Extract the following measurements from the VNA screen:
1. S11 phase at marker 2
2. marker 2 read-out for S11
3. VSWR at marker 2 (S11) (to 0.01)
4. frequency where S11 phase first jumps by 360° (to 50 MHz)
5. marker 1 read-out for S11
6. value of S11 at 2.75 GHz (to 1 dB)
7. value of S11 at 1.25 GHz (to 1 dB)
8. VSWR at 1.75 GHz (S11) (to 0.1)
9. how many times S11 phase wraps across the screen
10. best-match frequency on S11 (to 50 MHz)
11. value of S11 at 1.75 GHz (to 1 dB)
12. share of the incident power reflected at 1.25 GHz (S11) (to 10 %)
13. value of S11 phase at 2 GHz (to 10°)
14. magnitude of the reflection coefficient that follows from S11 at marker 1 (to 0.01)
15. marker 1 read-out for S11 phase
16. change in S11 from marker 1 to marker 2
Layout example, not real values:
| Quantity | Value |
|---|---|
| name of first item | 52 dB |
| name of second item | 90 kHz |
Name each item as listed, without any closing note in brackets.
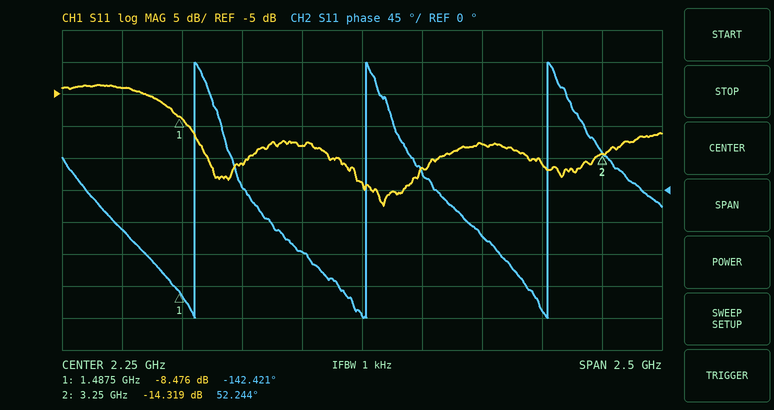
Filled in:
| Quantity | Value |
|---|---|
| S11 phase at marker 2 | 52.244° |
| marker 2 read-out for S11 | -14.319 dB |
| VSWR at marker 2 (S11) | 1.48 |
| frequency where S11 phase first jumps by 360° | 1.55 GHz |
| marker 1 read-out for S11 | -8.476 dB |
| value of S11 at 2.75 GHz | -13 dB |
| value of S11 at 1.25 GHz | -4 dB |
| VSWR at 1.75 GHz (S11) | 1.4 |
| how many times S11 phase wraps across the screen | 3 |
| best-match frequency on S11 | 2.35 GHz |
| value of S11 at 1.75 GHz | -16 dB |
| share of the incident power reflected at 1.25 GHz (S11) | 40 % |
| value of S11 phase at 2 GHz | -90° |
| magnitude of the reflection coefficient that follows from S11 at marker 1 | 0.38 |
| marker 1 read-out for S11 phase | -142.421° |
| change in S11 from marker 1 to marker 2 | -5.843 dB |
